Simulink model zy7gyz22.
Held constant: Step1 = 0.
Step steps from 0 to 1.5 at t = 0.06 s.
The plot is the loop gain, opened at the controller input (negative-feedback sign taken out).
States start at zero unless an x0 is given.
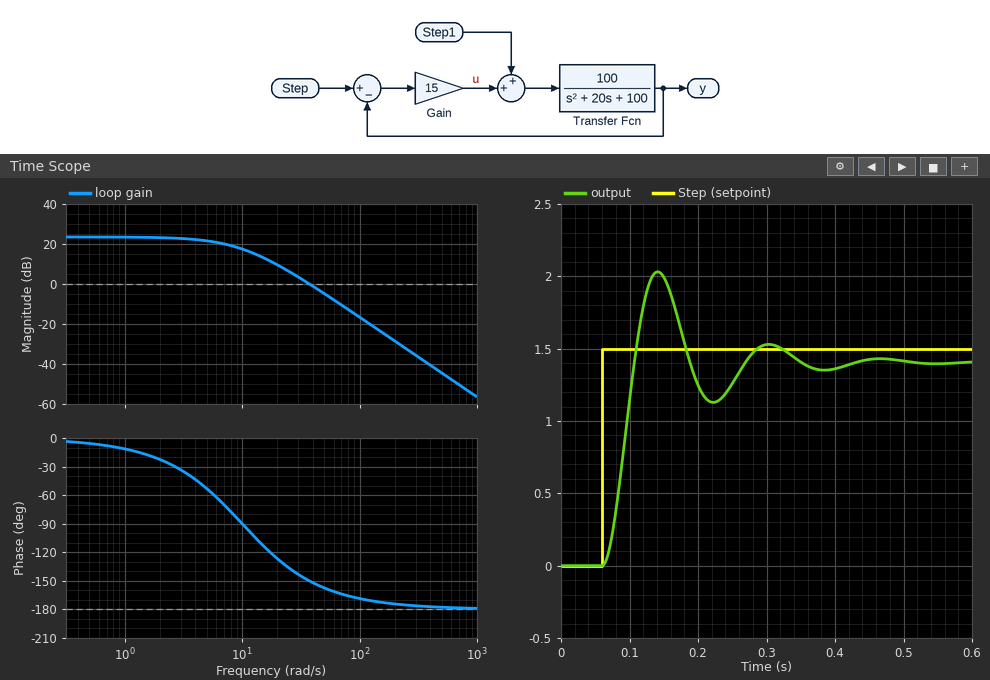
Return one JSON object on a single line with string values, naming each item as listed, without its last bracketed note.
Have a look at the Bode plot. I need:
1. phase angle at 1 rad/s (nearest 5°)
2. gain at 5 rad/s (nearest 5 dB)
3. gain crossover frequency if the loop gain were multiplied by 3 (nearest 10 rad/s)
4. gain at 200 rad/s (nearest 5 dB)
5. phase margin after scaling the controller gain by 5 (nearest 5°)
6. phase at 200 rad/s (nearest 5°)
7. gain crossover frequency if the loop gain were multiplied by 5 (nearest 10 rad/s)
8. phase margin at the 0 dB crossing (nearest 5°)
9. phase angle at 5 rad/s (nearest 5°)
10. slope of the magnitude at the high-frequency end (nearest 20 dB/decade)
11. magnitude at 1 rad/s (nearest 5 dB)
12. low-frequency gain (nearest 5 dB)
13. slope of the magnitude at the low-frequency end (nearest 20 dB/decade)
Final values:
{"phase angle at 1 rad/s": "-10°", "gain at 5 rad/s": "20 dB", "gain crossover frequency if the loop gain were multiplied by 3": "70 rad/s", "gain at 200 rad/s": "-30 dB", "phase margin after scaling the controller gain by 5": "15°", "phase at 200 rad/s": "-175°", "gain crossover frequency if the loop gain were multiplied by 5": "90 rad/s", "phase margin at the 0 dB crossing": "30°", "phase angle at 5 rad/s": "-55°", "slope of the magnitude at the high-frequency end": "-40 dB/decade", "magnitude at 1 rad/s": "25 dB", "low-frequency gain": "25 dB", "slope of the magnitude at the low-frequency end": "0 dB/decade"}
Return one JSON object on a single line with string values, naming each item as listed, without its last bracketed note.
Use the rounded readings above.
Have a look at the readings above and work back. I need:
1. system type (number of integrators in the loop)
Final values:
{"system type": "0"}
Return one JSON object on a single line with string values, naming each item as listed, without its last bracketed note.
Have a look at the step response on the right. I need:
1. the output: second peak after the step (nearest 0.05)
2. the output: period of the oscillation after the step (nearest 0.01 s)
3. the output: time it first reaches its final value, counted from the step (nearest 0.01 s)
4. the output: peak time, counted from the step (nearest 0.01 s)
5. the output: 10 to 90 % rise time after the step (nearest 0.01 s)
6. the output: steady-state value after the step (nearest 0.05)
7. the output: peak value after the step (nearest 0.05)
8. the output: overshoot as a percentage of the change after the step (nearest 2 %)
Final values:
{"the output: second peak after the step": "1.55", "the output: period of the oscillation after the step": "0.16 s", "the output: time it first reaches its final value, counted from the step": "0.05 s", "the output: peak time, counted from the step": "0.08 s", "the output: 10 to 90 % rise time after the step": "0.03 s", "the output: steady-state value after the step": "1.40", "the output: peak value after the step": "2.05", "the output: overshoot as a percentage of the change after the step": "44 %"}
